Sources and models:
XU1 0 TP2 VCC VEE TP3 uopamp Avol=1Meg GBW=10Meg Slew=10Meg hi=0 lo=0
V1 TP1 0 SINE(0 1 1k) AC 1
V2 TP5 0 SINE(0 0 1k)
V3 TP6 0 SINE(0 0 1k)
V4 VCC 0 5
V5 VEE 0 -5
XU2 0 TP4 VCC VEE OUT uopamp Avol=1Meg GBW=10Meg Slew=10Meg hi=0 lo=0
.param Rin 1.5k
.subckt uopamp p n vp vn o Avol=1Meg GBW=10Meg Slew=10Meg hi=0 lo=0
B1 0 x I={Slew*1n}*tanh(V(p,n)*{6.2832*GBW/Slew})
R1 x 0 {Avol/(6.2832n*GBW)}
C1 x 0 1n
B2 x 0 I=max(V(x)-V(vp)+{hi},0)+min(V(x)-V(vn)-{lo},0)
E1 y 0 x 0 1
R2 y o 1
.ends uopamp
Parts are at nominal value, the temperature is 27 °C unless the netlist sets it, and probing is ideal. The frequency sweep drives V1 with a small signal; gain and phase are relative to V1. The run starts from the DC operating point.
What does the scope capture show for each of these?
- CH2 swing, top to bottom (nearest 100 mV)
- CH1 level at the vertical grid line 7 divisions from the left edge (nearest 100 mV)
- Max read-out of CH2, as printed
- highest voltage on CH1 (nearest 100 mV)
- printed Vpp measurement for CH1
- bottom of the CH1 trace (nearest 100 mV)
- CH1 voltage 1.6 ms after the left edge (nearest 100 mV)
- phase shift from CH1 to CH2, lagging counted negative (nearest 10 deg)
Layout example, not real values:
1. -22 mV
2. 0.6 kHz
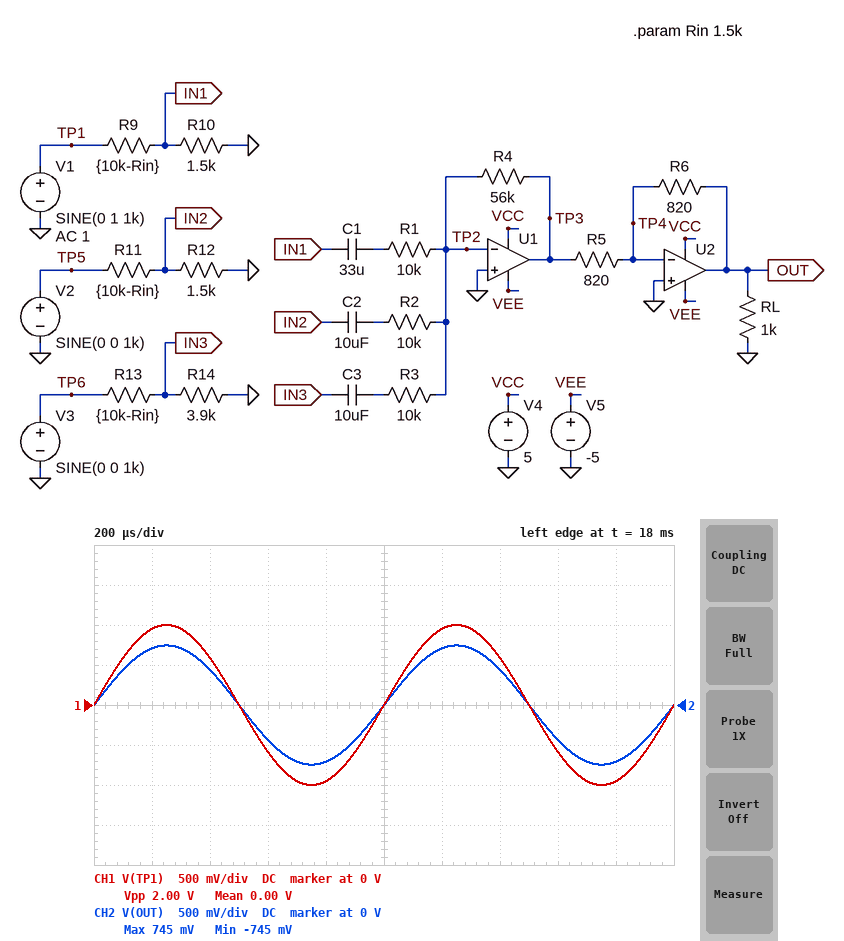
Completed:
1. 1.5 V
2. 600 mV
3. 745 mV
4. 1.0 V
5. 2.00 V
6. -1.0 V
7. -600 mV
8. 0 deg
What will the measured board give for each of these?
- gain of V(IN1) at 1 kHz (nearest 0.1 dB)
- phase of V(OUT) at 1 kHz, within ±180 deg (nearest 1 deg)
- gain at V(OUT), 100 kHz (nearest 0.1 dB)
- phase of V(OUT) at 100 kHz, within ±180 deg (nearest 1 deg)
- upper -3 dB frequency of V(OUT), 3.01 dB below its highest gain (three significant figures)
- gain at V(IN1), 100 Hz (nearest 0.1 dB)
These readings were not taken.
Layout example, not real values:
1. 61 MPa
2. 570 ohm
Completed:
1. -17.5 dB
2. 0 deg
3. -2.7 dB
4. -10 deg
5. 640 kHz
6. -17.5 dB
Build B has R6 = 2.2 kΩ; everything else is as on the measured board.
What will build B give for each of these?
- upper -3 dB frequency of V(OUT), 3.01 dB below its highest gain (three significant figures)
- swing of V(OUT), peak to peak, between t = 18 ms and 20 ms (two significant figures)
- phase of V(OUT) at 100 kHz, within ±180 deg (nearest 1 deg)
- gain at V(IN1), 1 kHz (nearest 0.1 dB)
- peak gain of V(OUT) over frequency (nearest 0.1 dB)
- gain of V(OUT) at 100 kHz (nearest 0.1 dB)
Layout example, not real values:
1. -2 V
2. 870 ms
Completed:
1. 618 kHz
2. 4.0 V
3. -11 deg
4. -17.5 dB
5. 6.0 dB
6. 5.9 dB
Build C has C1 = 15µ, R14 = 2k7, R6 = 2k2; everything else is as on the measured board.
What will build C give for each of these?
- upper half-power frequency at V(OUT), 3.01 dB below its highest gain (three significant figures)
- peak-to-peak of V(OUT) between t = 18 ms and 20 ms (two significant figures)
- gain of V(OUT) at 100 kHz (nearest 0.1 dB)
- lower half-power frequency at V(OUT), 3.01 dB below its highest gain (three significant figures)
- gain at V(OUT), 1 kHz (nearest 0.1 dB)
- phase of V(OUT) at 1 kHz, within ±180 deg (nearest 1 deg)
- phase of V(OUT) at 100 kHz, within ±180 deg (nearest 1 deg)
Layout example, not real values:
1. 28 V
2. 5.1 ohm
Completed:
1. 609 kHz
2. 4.0 V
3. 5.9 dB
4. 941 mHz
5. 6.0 dB
6. 0 deg
7. -11 deg
